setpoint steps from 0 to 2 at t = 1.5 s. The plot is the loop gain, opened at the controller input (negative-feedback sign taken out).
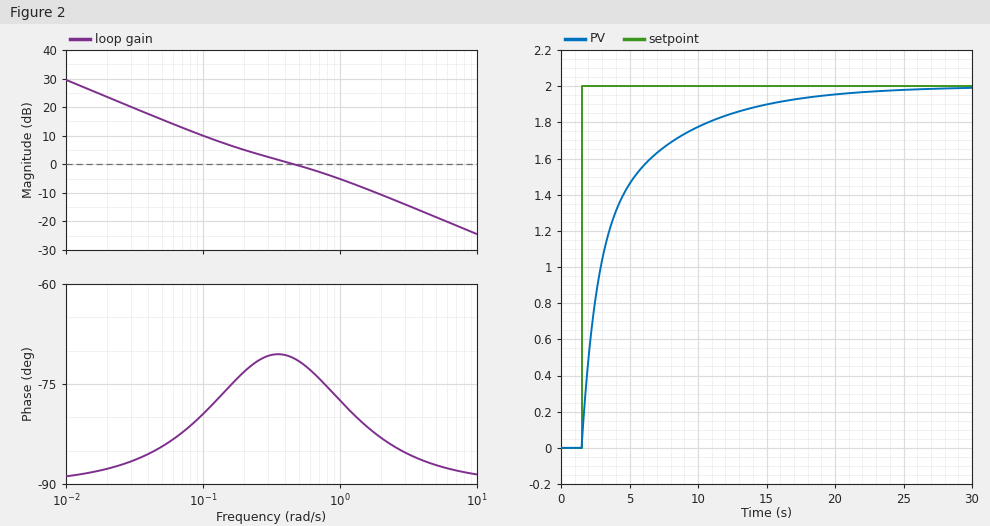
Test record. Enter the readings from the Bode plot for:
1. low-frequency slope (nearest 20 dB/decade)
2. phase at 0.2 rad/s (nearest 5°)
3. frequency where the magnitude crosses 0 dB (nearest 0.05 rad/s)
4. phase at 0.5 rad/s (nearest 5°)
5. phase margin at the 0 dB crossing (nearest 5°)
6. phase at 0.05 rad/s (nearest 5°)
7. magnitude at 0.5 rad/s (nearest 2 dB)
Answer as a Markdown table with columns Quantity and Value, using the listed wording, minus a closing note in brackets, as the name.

| Quantity | Value |
|---|---|
| low-frequency slope | -20 dB/decade |
| phase at 0.2 rad/s | -75° |
| frequency where the magnitude crosses 0 dB | 0.45 rad/s |
| phase at 0.5 rad/s | -70° |
| phase margin at the 0 dB crossing | 110° |
| phase at 0.05 rad/s | -85° |
| magnitude at 0.5 rad/s | 0 dB |
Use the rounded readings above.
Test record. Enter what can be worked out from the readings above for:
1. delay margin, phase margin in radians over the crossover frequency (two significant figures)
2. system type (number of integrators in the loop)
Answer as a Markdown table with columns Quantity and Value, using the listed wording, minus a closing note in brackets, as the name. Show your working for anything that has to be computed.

| Quantity | Value |
|---|---|
| delay margin, phase margin in radians over the crossover frequency | 110 × π / 180 / 0.45 = 4.3 s |
| system type | 1 |
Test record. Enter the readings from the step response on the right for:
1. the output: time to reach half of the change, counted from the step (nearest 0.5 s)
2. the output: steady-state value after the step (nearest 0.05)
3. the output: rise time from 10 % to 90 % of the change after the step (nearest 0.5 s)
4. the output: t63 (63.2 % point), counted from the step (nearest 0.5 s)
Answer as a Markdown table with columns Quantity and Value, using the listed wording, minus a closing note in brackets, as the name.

| Quantity | Value |
|---|---|
| the output: time to reach half of the change, counted from the step | 1.5 s |
| the output: steady-state value after the step | 2.00 |
| the output: rise time from 10 % to 90 % of the change after the step | 9.0 s |
| the output: t63 (63.2 % point), counted from the step | 2.5 s |
